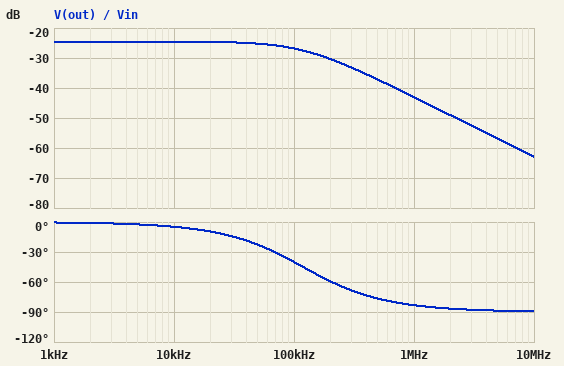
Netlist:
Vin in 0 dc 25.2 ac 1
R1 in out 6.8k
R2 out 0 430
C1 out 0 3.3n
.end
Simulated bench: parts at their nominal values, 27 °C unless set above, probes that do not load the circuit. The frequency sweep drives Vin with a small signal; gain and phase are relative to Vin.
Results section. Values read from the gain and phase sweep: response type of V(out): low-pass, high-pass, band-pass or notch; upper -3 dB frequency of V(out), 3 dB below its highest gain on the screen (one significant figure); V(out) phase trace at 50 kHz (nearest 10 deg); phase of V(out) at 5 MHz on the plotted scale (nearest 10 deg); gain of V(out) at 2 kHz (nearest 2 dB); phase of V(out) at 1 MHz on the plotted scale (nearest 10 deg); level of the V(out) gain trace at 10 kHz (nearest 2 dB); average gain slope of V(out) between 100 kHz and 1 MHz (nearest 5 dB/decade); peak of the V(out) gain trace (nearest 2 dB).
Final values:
low-pass
100 kHz
-20 deg
-90 deg
-24 dB
-80 deg
-24 dB
-15 dB/decade
-24 dB
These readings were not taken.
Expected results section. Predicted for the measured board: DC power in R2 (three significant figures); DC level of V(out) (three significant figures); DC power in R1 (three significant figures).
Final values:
5.22 mW
1.50 V
82.6 mW
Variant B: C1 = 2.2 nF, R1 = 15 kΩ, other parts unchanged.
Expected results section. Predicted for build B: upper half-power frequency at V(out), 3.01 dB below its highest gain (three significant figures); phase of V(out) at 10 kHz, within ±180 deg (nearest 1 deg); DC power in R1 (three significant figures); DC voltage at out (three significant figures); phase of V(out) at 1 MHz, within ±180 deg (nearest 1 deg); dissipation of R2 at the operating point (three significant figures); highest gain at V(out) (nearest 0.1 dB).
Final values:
173 kHz
-3 deg
40.0 mW
702 mV
-80 deg
1.15 mW
-31.1 dB
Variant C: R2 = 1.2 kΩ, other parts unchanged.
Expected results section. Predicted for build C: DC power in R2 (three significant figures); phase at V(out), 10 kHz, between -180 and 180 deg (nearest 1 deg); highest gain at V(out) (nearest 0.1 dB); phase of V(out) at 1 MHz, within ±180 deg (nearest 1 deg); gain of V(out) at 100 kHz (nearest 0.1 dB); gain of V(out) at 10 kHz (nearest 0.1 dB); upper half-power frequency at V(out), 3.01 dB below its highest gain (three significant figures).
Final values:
11.9 mW
-12 deg
-16.5 dB
-87 deg
-23.9 dB
-16.7 dB
47.3 kHz
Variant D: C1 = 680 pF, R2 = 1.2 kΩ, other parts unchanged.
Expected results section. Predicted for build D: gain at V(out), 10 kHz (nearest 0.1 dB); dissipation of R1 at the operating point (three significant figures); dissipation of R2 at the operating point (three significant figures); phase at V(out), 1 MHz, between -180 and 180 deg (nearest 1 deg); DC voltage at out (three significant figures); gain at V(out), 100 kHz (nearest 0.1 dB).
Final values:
-16.5 dB
67.5 mW
11.9 mW
-77 deg
3.78 V
-17.2 dB
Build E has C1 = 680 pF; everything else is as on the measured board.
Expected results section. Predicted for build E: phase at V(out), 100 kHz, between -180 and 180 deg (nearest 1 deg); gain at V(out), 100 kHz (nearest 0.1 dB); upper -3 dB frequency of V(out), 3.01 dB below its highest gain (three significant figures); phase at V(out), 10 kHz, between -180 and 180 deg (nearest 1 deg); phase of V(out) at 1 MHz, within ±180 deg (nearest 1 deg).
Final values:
-10 deg
-24.6 dB
579 kHz
-1 deg
-60 deg
